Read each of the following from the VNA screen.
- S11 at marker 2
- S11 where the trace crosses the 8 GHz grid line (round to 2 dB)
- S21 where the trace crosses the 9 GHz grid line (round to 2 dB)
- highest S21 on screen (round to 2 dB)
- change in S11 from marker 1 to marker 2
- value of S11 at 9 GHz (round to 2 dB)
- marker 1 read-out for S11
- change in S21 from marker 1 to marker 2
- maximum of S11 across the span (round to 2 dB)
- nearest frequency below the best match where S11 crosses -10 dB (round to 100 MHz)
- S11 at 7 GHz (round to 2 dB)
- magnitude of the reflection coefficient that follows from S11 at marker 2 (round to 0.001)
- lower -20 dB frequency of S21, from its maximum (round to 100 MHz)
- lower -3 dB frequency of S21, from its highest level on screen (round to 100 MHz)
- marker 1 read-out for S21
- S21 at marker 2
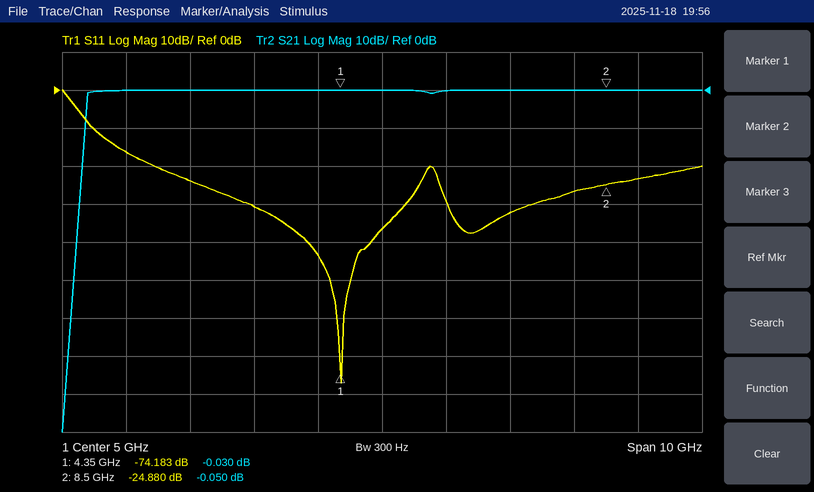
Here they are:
-24.880 dB
-26 dB
0 dB
0 dB
49.303 dB
-24 dB
-74.183 dB
-0.020 dB
0 dB
500 MHz
-32 dB
0.057
300 MHz
400 MHz
-0.030 dB
-0.050 dB
